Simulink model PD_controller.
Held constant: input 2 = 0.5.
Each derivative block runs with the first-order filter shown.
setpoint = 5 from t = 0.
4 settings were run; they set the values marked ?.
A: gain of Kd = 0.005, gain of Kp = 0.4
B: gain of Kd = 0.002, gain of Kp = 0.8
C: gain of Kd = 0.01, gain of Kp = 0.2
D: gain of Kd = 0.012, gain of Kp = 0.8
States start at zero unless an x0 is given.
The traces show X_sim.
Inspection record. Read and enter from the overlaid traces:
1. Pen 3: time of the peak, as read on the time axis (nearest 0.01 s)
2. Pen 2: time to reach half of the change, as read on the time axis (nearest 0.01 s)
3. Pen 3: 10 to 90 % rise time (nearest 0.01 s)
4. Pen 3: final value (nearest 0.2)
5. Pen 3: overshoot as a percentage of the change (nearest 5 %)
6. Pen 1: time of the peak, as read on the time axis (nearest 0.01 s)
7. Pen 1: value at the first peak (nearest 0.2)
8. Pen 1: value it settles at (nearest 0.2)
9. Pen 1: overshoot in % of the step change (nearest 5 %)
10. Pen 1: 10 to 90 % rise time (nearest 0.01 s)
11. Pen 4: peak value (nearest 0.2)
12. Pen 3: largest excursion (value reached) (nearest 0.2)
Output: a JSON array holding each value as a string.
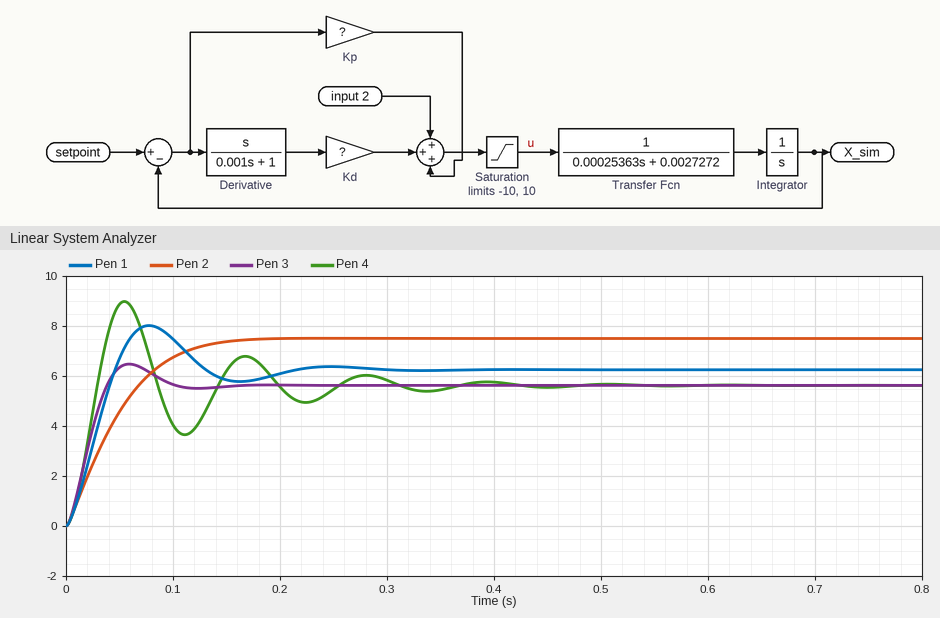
["0.06 s", "0.04 s", "0.03 s", "5.6", "15 %", "0.08 s", "8.0", "6.2", "30 %", "0.03 s", "9.0", "6.4"]
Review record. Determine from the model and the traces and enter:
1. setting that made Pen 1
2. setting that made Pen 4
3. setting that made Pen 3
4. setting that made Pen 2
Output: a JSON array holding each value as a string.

["A", "B", "D", "C"]
